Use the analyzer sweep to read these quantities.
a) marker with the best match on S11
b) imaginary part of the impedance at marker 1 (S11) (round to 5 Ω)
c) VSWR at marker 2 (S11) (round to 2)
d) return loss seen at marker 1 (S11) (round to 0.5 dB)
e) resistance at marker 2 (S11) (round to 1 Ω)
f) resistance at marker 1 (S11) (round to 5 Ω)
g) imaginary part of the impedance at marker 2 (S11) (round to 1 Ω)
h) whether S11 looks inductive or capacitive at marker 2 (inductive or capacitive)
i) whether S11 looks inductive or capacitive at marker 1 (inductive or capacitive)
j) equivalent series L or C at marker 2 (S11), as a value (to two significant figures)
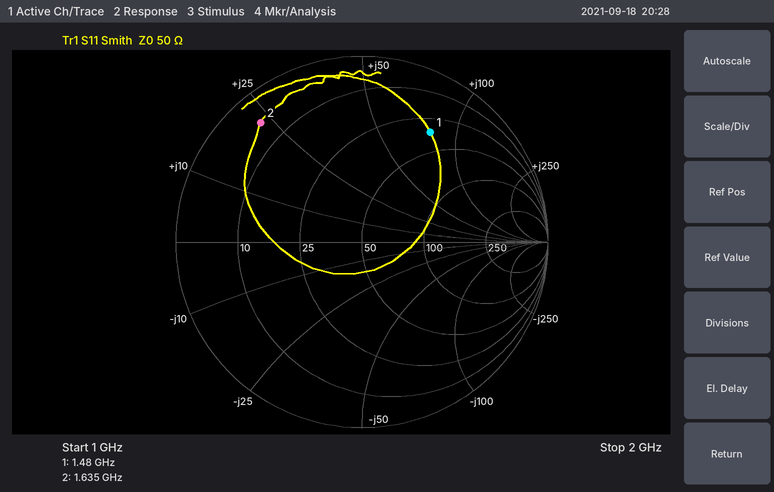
marker 1
+80 Ω
12
3.0 dB
5 Ω
35 Ω
+23 Ω
inductive
inductive
2.2 nH
